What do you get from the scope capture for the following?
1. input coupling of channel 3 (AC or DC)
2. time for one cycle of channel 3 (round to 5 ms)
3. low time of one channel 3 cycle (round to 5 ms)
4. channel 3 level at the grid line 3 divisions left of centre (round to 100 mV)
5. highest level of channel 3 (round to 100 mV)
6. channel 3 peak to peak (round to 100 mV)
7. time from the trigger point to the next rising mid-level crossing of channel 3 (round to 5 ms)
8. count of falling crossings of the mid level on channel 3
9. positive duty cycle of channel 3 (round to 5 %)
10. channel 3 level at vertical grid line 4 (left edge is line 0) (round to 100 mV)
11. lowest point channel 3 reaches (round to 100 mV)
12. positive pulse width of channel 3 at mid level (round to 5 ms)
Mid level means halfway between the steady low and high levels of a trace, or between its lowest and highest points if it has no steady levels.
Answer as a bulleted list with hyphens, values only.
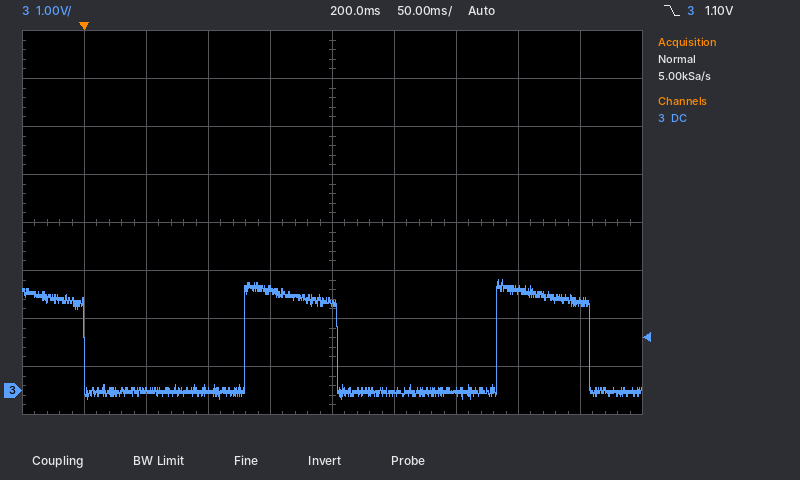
- DC
- 205 ms
- 130 ms
- 0.0 V
- 2.3 V
- 2.5 V
- 130 ms
- 3
- 35 %
- 2.1 V
- -200 mV
- 75 ms
